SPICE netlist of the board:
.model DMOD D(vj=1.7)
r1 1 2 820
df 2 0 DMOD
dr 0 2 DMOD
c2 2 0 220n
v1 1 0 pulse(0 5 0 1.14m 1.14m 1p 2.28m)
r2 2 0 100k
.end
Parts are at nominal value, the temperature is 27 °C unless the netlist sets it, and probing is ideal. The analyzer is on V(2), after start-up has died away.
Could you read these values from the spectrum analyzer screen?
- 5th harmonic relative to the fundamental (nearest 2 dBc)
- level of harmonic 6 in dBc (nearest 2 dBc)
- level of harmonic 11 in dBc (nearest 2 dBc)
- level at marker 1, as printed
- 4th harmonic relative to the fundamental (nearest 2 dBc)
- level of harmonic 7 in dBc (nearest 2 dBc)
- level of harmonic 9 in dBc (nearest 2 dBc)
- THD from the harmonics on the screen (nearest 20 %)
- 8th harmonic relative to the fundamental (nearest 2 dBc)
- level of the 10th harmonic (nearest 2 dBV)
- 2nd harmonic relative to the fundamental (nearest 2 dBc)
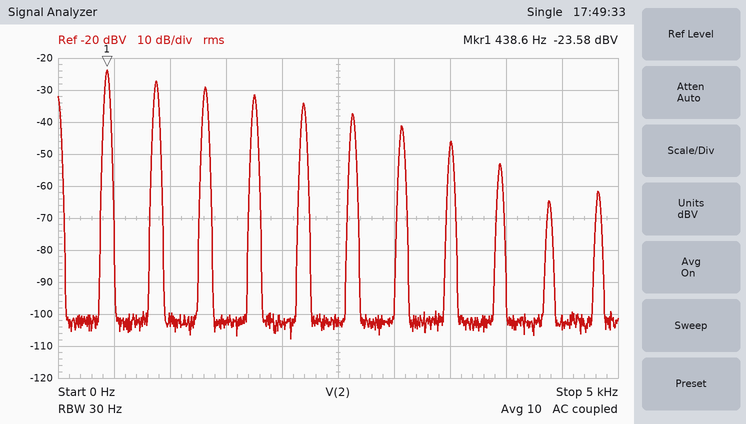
-10 dBc
-14 dBc
-38 dBc
-23.58 dBV
-8 dBc
-18 dBc
-30 dBc
100 %
-22 dBc
-64 dBV
-4 dBc
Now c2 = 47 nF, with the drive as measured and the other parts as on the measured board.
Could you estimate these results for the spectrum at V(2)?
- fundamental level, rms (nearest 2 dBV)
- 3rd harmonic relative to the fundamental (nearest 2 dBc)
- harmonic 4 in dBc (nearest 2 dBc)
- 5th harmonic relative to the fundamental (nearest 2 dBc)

-22 dBV
-4 dBc
-6 dBc
-8 dBc
